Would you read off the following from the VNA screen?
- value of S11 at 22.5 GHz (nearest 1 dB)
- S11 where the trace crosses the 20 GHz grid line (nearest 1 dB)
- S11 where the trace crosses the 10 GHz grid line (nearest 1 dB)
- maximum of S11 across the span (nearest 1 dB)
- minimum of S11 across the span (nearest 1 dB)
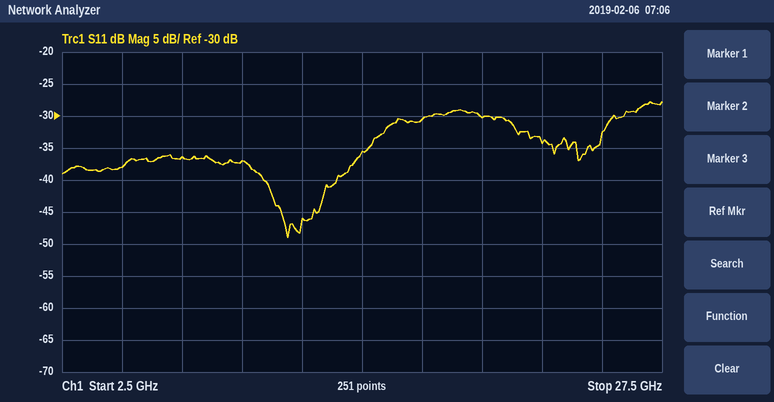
-34 dB
-30 dB
-37 dB
-28 dB
-49 dB
